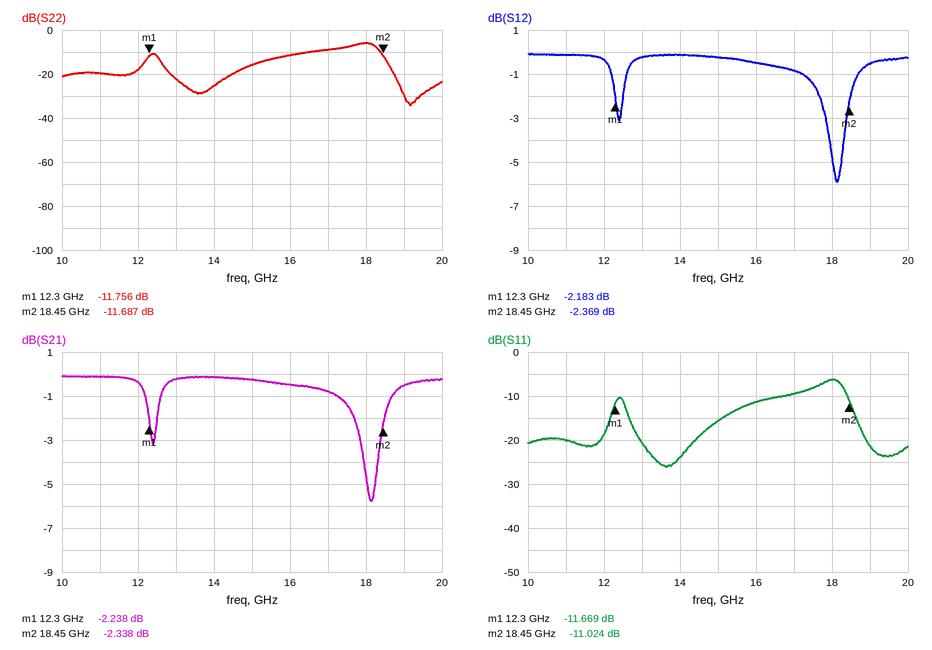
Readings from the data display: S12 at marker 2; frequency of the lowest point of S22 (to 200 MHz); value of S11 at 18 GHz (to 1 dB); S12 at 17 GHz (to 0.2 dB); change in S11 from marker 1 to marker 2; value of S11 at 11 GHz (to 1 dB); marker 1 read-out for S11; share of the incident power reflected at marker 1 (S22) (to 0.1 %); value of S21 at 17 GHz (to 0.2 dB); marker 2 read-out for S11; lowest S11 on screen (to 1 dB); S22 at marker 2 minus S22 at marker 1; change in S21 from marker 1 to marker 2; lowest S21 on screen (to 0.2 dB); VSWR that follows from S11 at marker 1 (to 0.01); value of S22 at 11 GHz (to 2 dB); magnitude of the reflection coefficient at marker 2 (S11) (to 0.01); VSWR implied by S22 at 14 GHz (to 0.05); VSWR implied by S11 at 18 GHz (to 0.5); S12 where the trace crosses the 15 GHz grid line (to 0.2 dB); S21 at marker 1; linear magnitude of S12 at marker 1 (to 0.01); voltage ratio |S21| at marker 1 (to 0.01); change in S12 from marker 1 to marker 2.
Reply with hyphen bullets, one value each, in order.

- -2.369 dB
- 19.2 GHz
- -6 dB
- -0.8 dB
- 0.645 dB
- -20 dB
- -11.669 dB
- 6.7 %
- -0.8 dB
- -11.024 dB
- -26 dB
- 0.069 dB
- -0.100 dB
- -5.8 dB
- 1.71
- -20 dB
- 0.28
- 1.10
- 3.0
- -0.2 dB
- -2.238 dB
- 0.78
- 0.77
- -0.186 dB
